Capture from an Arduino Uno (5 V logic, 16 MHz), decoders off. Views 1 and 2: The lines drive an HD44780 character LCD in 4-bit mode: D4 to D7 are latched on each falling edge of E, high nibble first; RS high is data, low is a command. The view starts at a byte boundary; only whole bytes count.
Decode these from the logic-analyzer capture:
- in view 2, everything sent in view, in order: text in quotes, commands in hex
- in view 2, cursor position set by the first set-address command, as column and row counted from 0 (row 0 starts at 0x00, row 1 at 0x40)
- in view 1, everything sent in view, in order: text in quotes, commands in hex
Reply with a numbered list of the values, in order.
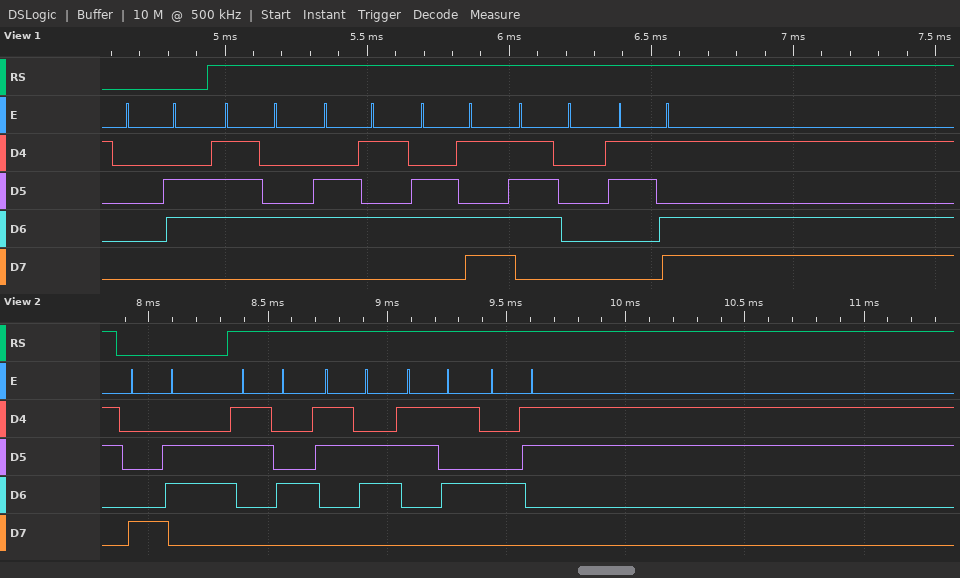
1. 0x86 "465C"
2. column 6, row 0
3. 0x06 "temp="
